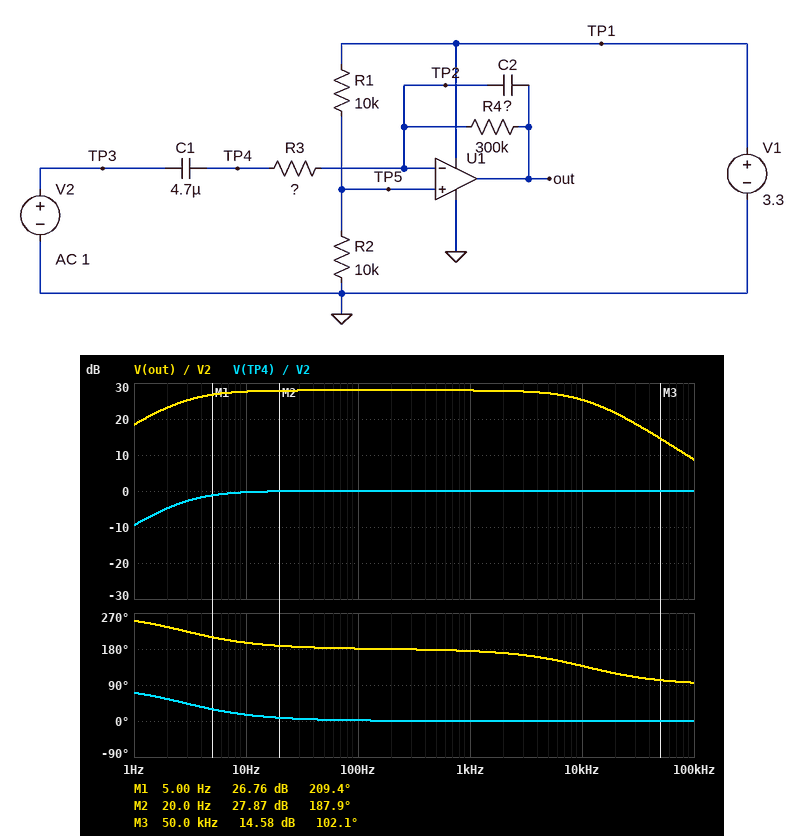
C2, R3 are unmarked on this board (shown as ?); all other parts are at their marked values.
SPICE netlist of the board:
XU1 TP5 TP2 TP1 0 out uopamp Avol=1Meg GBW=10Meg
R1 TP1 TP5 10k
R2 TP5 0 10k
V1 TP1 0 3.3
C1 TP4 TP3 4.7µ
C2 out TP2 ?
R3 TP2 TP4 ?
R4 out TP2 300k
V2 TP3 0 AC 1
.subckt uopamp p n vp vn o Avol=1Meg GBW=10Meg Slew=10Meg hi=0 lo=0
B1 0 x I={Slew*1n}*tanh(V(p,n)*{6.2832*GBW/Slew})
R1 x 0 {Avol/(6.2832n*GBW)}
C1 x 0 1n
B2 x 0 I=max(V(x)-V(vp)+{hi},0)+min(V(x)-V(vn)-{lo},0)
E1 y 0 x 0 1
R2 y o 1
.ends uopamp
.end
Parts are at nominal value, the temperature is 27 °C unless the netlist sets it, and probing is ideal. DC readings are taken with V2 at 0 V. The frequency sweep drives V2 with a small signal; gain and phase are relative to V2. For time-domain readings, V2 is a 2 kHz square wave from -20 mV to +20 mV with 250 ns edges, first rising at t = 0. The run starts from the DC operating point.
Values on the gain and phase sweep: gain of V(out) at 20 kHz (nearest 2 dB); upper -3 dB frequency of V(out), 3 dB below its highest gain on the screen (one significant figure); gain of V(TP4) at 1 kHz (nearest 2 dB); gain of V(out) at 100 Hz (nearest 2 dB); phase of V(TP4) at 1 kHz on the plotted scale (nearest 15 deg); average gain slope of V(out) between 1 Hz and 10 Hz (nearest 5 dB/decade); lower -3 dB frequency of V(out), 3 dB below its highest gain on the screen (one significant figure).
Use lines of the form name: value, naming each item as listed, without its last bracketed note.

gain of V(out) at 20 kHz: 22 dB
upper -3 dB frequency of V(out), 3 dB below its highest gain on the screen: 10 kHz
gain of V(TP4) at 1 kHz: 0 dB
gain of V(out) at 100 Hz: 28 dB
phase of V(TP4) at 1 kHz on the plotted scale: 0 deg
average gain slope of V(out) between 1 Hz and 10 Hz: 10 dB/decade
lower -3 dB frequency of V(out), 3 dB below its highest gain on the screen: 3 Hz
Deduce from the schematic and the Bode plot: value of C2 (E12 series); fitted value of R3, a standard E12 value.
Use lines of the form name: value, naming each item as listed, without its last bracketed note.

value of C2: 47 pF
fitted value of R3, a standard E12 value: 12 kΩ
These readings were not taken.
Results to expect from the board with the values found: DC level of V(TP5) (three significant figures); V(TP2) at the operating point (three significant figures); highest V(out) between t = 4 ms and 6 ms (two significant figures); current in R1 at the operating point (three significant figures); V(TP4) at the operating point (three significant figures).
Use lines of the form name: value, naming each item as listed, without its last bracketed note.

DC level of V(TP5): 1.65 V
V(TP2) at the operating point: 1.65 V
highest V(out) between t = 4 ms and 6 ms: 1.7 V
current in R1 at the operating point: 165 µA
V(TP4) at the operating point: 1.65 V
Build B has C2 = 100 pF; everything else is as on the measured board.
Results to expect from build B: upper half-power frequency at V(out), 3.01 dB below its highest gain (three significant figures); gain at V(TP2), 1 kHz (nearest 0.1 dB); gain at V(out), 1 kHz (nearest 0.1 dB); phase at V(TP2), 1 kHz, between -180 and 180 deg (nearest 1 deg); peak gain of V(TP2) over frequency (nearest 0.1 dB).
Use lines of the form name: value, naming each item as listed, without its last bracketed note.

upper half-power frequency at V(out), 3.01 dB below its highest gain: 5.24 kHz
gain at V(TP2), 1 kHz: -52.2 dB
gain at V(out), 1 kHz: 27.8 dB
phase at V(TP2), 1 kHz, between -180 and 180 deg: 79 deg
peak gain of V(TP2) over frequency: -37.7 dB
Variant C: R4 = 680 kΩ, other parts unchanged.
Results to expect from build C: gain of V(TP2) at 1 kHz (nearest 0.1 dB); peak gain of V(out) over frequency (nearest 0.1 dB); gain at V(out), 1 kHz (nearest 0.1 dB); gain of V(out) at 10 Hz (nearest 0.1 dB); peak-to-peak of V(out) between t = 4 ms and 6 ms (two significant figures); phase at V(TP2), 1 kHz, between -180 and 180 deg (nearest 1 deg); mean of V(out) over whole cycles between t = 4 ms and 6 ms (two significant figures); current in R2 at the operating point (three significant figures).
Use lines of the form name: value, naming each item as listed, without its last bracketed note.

gain of V(TP2) at 1 kHz: -45.1 dB
peak gain of V(out) over frequency: 35.1 dB
gain at V(out), 1 kHz: 34.9 dB
gain of V(out) at 10 Hz: 34.7 dB
peak-to-peak of V(out) between t = 4 ms and 6 ms: 1.7 V
phase at V(TP2), 1 kHz, between -180 and 180 deg: 78 deg
mean of V(out) over whole cycles between t = 4 ms and 6 ms: 810 mV
current in R2 at the operating point: 165 µA
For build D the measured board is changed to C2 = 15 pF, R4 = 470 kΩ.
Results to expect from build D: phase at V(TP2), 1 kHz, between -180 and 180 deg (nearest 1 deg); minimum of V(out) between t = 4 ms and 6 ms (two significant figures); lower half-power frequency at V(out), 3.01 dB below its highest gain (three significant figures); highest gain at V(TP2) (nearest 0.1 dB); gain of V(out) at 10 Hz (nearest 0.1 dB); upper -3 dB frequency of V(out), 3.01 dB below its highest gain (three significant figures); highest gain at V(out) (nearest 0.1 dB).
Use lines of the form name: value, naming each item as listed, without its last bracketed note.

phase at V(TP2), 1 kHz, between -180 and 180 deg: 87 deg
minimum of V(out) between t = 4 ms and 6 ms: 140 mV
lower half-power frequency at V(out), 3.01 dB below its highest gain: 2.82 Hz
highest gain at V(TP2): -21.8 dB
gain of V(out) at 10 Hz: 31.5 dB
upper -3 dB frequency of V(out), 3.01 dB below its highest gain: 20.7 kHz
highest gain at V(out): 31.9 dB
